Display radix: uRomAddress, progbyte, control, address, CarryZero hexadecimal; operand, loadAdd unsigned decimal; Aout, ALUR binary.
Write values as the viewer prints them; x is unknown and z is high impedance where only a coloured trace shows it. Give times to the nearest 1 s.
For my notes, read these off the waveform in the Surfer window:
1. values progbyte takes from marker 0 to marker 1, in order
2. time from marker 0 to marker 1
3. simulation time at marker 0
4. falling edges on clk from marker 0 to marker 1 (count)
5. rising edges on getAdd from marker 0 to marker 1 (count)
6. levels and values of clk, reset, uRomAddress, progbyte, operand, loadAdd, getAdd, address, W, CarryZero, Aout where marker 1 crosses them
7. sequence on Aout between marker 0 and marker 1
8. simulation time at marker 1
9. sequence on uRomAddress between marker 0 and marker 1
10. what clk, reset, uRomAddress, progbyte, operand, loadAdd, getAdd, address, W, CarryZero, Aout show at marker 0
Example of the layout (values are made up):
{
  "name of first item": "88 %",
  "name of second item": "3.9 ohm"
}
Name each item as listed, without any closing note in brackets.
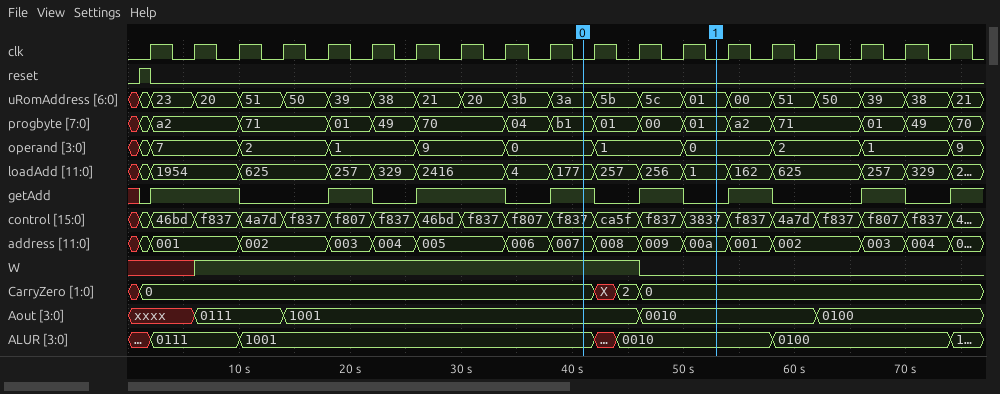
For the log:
{
  "values progbyte takes from marker 0 to marker 1, in order": "b1, 01, 00, 01",
  "time from marker 0 to marker 1": "12 s",
  "simulation time at marker 0": "41 s",
  "falling edges on clk from marker 0 to marker 1": "3",
  "rising edges on getAdd from marker 0 to marker 1": "1",
  "levels and values of clk, reset, uRomAddress, progbyte, operand, loadAdd, getAdd, address, W, CarryZero, Aout where marker 1 crosses them": "clk=0, reset=0, uRomAddress=01, progbyte=01, operand=0, loadAdd=1, getAdd=0, address=00a, W=0, CarryZero=0, Aout=0010",
  "sequence on Aout between marker 0 and marker 1": "1001, 0010",
  "simulation time at marker 1": "53 s",
  "sequence on uRomAddress between marker 0 and marker 1": "3a, 5b, 5c, 01",
  "what clk, reset, uRomAddress, progbyte, operand, loadAdd, getAdd, address, W, CarryZero, Aout show at marker 0": "clk=0, reset=0, uRomAddress=3a, progbyte=b1, operand=0, loadAdd=177, getAdd=1, address=007, W=1, CarryZero=0, Aout=1001"
}
